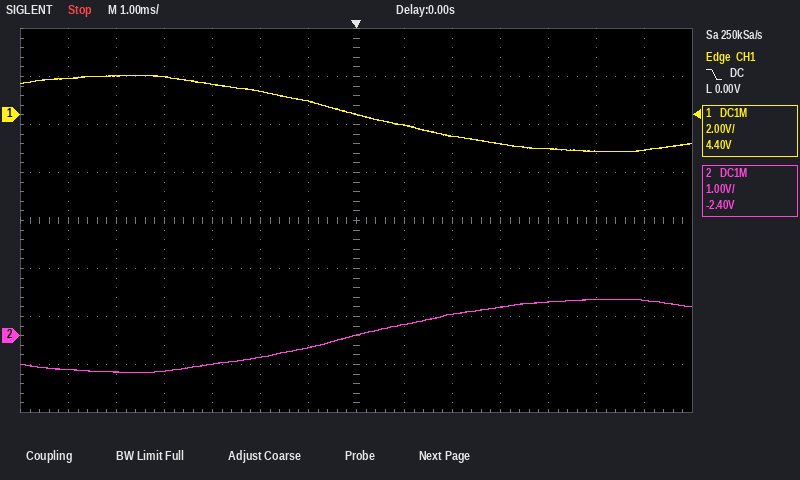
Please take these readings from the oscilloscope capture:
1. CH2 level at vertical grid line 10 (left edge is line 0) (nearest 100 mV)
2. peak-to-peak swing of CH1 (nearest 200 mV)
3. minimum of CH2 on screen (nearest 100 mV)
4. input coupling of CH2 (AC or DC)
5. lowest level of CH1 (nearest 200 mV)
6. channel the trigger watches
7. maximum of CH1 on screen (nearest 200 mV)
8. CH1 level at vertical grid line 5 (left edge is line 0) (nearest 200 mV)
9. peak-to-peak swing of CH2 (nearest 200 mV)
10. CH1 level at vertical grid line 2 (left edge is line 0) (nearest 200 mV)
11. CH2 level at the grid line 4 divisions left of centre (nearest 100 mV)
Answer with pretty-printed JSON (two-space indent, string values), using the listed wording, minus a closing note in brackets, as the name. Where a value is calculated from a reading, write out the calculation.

{
  "CH2 level at vertical grid line 10 (left edge is line 0)": "600 mV",
  "peak-to-peak swing of CH1": "1.6 V − (-1.6 V) = 3.2 V",
  "minimum of CH2 on screen": "-800 mV",
  "input coupling of CH2": "DC",
  "lowest level of CH1": "-1.6 V",
  "channel the trigger watches": "CH1",
  "maximum of CH1 on screen": "1.6 V",
  "CH1 level at vertical grid line 5 (left edge is line 0)": "1.0 V",
  "peak-to-peak swing of CH2": "1.6 V",
  "CH1 level at vertical grid line 2 (left edge is line 0)": "1.6 V",
  "CH2 level at the grid line 4 divisions left of centre": "-700 mV"
}
